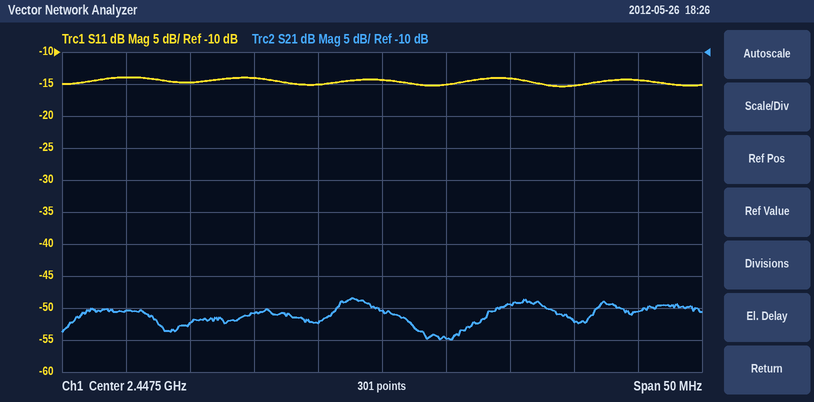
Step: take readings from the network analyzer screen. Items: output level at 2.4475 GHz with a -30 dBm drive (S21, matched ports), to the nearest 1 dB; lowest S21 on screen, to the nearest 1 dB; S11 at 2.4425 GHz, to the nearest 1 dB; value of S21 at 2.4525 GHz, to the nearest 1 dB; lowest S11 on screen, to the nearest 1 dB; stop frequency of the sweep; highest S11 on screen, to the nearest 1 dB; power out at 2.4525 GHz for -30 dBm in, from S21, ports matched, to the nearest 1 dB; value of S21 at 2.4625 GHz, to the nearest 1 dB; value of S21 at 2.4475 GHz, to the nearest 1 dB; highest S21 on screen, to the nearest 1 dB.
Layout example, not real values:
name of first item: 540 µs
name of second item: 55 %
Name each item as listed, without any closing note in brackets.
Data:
output level at 2.4475 GHz with a -30 dBm drive (S21, matched ports), to the nearest 1 dB: -80 dBm
lowest S21 on screen, to the nearest 1 dB: -55 dB
S11 at 2.4425 GHz, to the nearest 1 dB: -15 dB
value of S21 at 2.4525 GHz, to the nearest 1 dB: -55 dB
lowest S11 on screen, to the nearest 1 dB: -15 dB
stop frequency of the sweep: 2.4725 GHz
highest S11 on screen, to the nearest 1 dB: -14 dB
power out at 2.4525 GHz for -30 dBm in, from S21, ports matched, to the nearest 1 dB: -85 dBm
value of S21 at 2.4625 GHz, to the nearest 1 dB: -52 dB
value of S21 at 2.4475 GHz, to the nearest 1 dB: -50 dB
highest S21 on screen, to the nearest 1 dB: -48 dB
